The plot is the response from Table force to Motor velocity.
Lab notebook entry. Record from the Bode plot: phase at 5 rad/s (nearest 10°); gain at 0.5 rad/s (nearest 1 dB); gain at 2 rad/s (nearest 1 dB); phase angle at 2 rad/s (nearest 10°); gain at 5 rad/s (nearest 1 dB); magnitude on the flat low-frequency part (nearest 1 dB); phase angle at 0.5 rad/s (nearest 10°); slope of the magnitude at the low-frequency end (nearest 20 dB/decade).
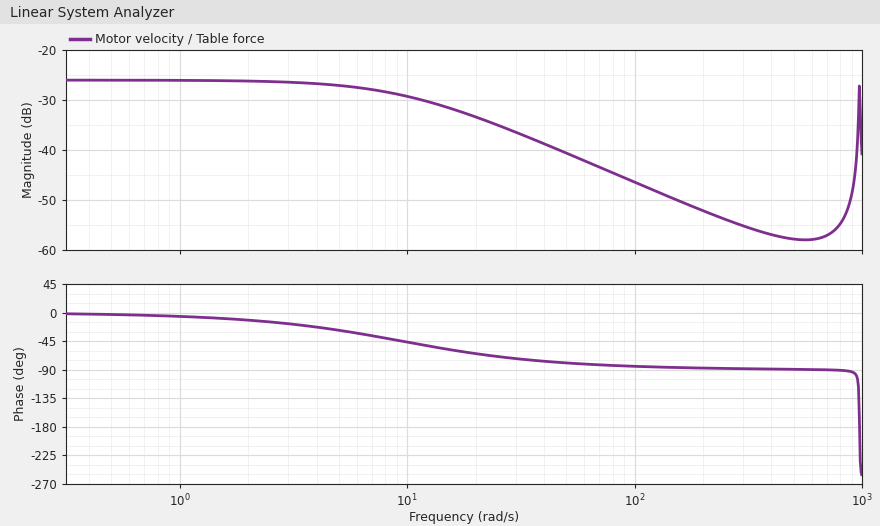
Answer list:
-30°
-26 dB
-26 dB
-10°
-27 dB
-26 dB
0°
0 dB/decade
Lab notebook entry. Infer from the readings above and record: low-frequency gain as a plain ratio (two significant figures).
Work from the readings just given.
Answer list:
0.050
